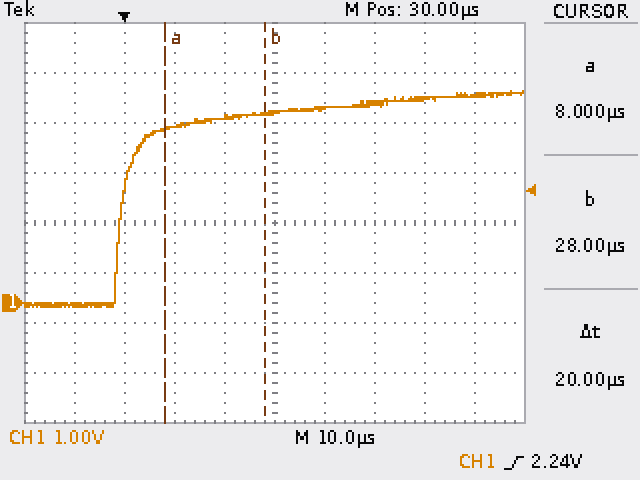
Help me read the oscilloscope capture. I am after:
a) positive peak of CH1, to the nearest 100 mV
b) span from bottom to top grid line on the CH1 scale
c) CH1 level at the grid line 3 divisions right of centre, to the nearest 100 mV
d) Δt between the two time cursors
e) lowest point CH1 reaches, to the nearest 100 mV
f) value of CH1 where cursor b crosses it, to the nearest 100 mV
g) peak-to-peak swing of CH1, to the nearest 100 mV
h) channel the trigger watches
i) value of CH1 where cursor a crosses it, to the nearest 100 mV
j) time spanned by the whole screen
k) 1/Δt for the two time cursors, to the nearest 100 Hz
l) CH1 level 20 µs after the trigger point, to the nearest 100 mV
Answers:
4.2 V
8 V
4.1 V
20 µs
-100 mV
3.8 V
4.3 V
CH1
3.5 V
100 µs
50.0 kHz
3.7 V
